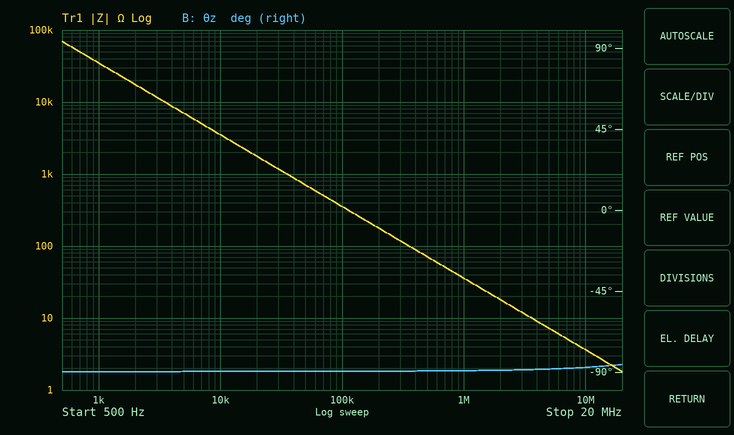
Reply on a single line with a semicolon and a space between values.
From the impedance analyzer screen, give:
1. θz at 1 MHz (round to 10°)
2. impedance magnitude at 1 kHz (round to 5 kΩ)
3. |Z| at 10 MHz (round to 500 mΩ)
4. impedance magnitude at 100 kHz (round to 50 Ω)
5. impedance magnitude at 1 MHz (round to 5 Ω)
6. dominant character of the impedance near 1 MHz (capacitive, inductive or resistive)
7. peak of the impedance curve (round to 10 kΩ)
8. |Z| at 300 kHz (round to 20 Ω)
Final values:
-90°; 35 kΩ; 3.5 Ω; 350 Ω; 35 Ω; capacitive; 70 kΩ; 120 Ω
